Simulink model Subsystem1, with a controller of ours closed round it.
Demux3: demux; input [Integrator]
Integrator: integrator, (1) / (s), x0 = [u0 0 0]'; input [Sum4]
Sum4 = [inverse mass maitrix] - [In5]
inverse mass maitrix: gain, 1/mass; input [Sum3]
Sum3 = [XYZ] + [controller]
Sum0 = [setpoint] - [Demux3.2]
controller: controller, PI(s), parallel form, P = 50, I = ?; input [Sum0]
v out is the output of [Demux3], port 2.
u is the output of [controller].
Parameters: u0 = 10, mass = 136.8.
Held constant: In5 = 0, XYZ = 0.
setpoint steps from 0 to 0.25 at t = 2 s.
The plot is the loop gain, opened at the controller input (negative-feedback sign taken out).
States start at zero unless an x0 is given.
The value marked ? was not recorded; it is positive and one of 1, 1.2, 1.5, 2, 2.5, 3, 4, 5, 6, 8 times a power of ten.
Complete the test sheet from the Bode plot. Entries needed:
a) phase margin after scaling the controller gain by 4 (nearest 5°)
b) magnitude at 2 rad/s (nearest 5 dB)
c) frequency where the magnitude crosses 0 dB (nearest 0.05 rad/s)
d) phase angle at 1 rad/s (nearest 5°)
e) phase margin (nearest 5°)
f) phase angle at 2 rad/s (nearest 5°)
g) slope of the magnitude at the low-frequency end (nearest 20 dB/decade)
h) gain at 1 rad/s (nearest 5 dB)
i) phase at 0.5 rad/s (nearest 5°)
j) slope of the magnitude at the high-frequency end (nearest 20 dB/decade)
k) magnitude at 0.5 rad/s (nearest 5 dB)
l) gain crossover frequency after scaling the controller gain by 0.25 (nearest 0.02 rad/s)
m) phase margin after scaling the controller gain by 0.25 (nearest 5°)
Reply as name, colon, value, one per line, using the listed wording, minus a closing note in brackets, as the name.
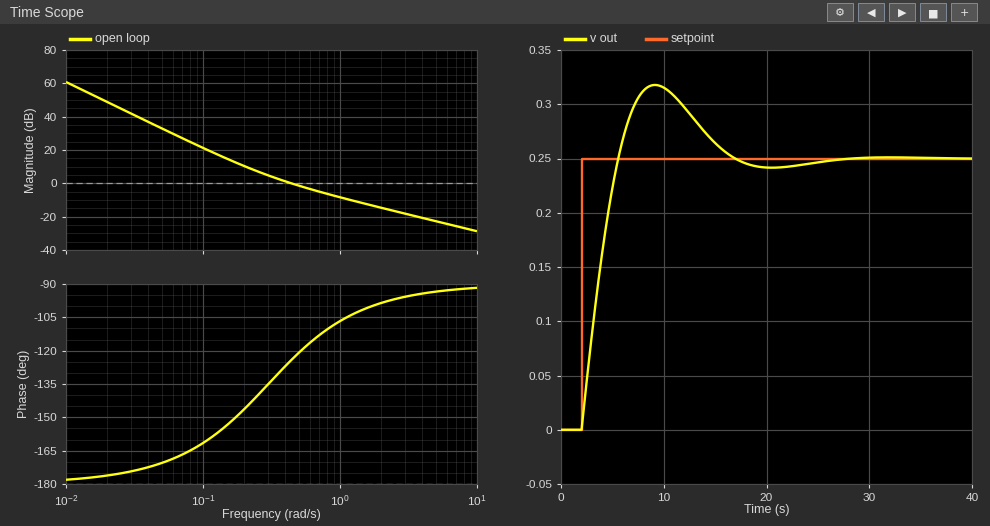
phase margin after scaling the controller gain by 4: 80°
magnitude at 2 rad/s: -15 dB
frequency where the magnitude crosses 0 dB: 0.45 rad/s
phase angle at 1 rad/s: -105°
phase margin: 55°
phase angle at 2 rad/s: -100°
slope of the magnitude at the low-frequency end: -40 dB/decade
gain at 1 rad/s: -10 dB
phase at 0.5 rad/s: -120°
slope of the magnitude at the high-frequency end: -20 dB/decade
magnitude at 0.5 rad/s: 0 dB
gain crossover frequency after scaling the controller gain by 0.25: 0.18 rad/s
phase margin after scaling the controller gain by 0.25: 30°
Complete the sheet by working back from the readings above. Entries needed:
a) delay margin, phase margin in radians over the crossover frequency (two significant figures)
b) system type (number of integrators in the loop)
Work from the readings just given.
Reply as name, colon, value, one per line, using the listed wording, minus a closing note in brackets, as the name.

delay margin, phase margin in radians over the crossover frequency: 2.1 s
system type: 2
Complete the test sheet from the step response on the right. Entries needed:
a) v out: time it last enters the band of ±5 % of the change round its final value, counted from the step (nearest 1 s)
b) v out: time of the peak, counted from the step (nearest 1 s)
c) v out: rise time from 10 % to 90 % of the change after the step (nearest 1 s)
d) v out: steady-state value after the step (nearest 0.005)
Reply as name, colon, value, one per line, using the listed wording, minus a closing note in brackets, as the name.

v out: time it last enters the band of ±5 % of the change round its final value, counted from the step: 13 s
v out: time of the peak, counted from the step: 7 s
v out: rise time from 10 % to 90 % of the change after the step: 3 s
v out: steady-state value after the step: 0.250
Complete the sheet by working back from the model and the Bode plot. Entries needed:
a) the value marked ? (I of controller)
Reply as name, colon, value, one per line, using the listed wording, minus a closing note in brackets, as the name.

the value marked ?: 15
